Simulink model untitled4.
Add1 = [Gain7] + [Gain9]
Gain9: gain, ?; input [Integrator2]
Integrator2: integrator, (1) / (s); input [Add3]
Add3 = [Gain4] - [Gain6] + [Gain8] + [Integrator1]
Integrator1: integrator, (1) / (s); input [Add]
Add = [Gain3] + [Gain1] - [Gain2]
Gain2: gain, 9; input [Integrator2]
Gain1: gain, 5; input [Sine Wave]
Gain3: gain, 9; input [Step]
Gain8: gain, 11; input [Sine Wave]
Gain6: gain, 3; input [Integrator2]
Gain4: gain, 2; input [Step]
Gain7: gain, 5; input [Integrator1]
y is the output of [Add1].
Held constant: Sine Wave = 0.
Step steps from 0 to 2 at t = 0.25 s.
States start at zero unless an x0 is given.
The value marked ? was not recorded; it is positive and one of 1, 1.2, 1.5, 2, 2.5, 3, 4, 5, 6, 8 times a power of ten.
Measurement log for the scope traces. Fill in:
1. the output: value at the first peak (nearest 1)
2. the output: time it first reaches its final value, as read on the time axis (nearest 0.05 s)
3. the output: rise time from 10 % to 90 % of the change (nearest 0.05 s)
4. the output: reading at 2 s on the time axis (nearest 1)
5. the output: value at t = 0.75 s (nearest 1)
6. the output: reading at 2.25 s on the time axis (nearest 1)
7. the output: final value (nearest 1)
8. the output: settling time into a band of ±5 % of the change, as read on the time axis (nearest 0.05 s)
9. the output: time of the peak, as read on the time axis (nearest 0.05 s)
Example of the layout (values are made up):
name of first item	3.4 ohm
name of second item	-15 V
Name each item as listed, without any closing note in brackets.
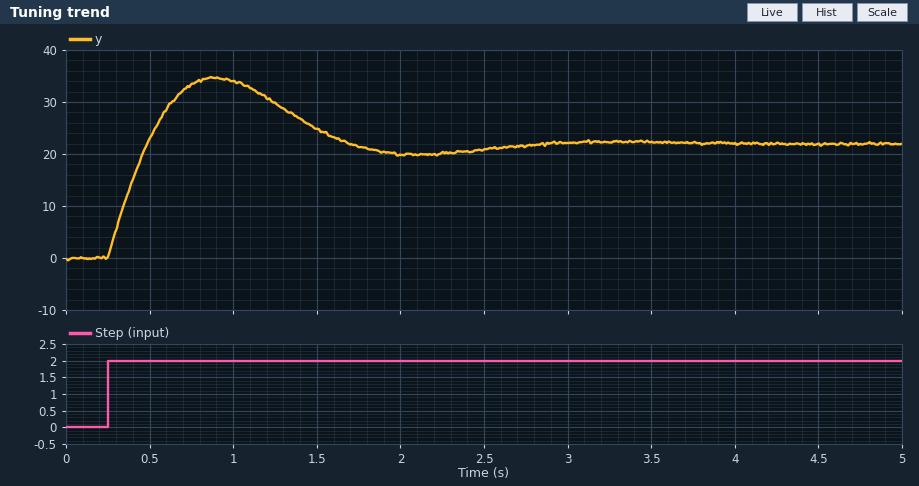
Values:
the output: value at the first peak	35
the output: time it first reaches its final value, as read on the time axis	0.50 s
the output: rise time from 10 % to 90 % of the change	0.20 s
the output: reading at 2 s on the time axis	20
the output: value at t = 0.75 s	33
the output: reading at 2.25 s on the time axis	20
the output: final value	22
the output: settling time into a band of ±5 % of the change, as read on the time axis	2.50 s
the output: time of the peak, as read on the time axis	0.90 s
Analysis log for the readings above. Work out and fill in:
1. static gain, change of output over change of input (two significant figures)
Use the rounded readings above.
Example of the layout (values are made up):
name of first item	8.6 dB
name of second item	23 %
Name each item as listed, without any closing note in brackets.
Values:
static gain, change of output over change of input	11
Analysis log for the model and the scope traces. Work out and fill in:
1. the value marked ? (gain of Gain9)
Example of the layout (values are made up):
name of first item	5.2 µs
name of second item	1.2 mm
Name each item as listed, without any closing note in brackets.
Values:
the value marked ?	6
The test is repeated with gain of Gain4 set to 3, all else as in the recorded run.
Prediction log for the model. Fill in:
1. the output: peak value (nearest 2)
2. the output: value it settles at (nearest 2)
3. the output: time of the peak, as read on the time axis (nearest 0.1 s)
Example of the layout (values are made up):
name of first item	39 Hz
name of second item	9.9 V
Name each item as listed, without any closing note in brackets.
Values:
the output: peak value	30
the output: value it settles at	12
the output: time of the peak, as read on the time axis	0.8 s
